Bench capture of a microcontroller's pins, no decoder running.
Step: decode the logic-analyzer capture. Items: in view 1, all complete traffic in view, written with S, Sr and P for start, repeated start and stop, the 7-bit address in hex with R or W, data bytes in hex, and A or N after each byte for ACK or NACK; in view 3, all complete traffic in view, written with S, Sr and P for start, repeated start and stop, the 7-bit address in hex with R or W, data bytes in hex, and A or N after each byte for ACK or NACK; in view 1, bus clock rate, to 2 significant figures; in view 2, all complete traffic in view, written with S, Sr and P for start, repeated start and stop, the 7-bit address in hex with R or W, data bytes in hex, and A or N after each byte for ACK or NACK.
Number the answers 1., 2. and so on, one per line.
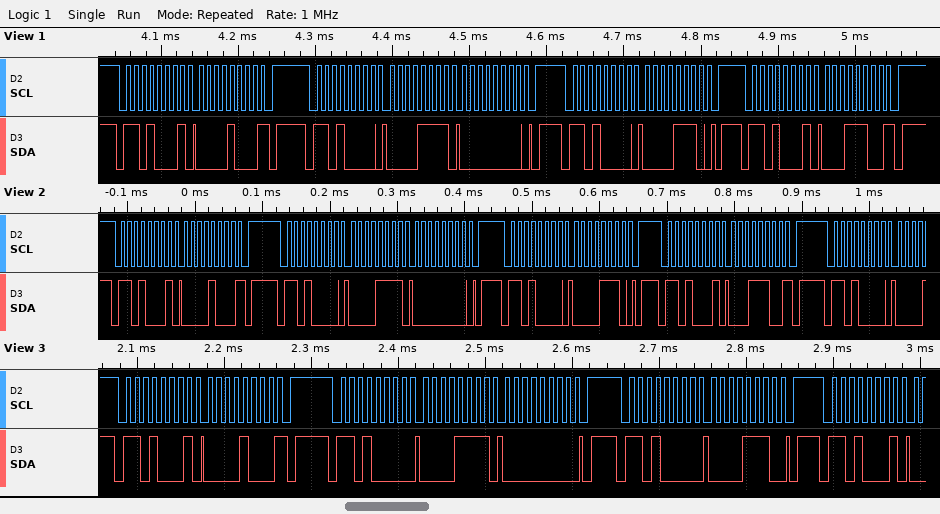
1. S 68R A 08 N P S 68W A 0F A 00 A P S 68W A 0E A P S 68R A 1C N P
2. S 68R A 08 N P S 68W A 0F A 00 A P S 68W A 0E A P S 68R A
3. 100 kHz
4. S 68R A 08 N P S 68W A 0F A 00 A P S 68W A 0E A P S 68R A 1C N P S 68W A
